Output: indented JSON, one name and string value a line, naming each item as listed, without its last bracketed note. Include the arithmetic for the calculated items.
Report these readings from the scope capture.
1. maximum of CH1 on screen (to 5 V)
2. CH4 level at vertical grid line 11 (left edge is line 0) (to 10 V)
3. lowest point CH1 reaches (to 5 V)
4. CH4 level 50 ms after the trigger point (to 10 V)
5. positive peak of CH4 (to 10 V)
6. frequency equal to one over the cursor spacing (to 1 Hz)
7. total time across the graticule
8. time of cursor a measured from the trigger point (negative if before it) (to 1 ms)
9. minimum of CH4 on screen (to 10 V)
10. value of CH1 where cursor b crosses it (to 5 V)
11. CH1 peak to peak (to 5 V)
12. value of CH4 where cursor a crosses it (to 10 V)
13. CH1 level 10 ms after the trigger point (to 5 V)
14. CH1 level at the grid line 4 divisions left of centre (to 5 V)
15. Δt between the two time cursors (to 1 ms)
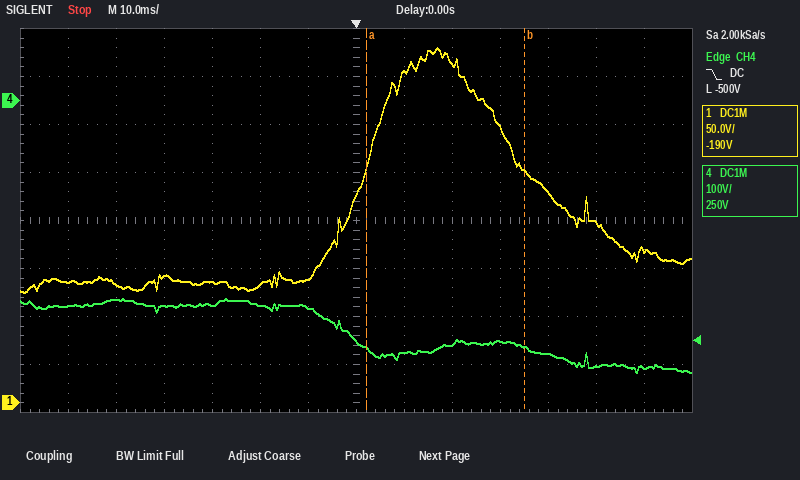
{
  "maximum of CH1 on screen": "370 V",
  "CH4 level at vertical grid line 11 (left edge is line 0)": "-530 V",
  "lowest point CH1 reaches": "115 V",
  "CH4 level 50 ms after the trigger point": "-550 V",
  "positive peak of CH4": "-410 V",
  "frequency equal to one over the cursor spacing": "1 / 33 ms ≈ 30 Hz",
  "total time across the graticule": "140 ms",
  "time of cursor a measured from the trigger point (negative if before it)": "+2 ms",
  "minimum of CH4 on screen": "-570 V",
  "value of CH1 where cursor b crosses it": "240 V",
  "CH1 peak to peak": "370 V − (115 V) = 255 V",
  "value of CH4 where cursor a crosses it": "-520 V",
  "CH1 level 10 ms after the trigger point": "345 V",
  "CH1 level at the grid line 4 divisions left of centre": "130 V",
  "Δt between the two time cursors": "33 ms"
}
